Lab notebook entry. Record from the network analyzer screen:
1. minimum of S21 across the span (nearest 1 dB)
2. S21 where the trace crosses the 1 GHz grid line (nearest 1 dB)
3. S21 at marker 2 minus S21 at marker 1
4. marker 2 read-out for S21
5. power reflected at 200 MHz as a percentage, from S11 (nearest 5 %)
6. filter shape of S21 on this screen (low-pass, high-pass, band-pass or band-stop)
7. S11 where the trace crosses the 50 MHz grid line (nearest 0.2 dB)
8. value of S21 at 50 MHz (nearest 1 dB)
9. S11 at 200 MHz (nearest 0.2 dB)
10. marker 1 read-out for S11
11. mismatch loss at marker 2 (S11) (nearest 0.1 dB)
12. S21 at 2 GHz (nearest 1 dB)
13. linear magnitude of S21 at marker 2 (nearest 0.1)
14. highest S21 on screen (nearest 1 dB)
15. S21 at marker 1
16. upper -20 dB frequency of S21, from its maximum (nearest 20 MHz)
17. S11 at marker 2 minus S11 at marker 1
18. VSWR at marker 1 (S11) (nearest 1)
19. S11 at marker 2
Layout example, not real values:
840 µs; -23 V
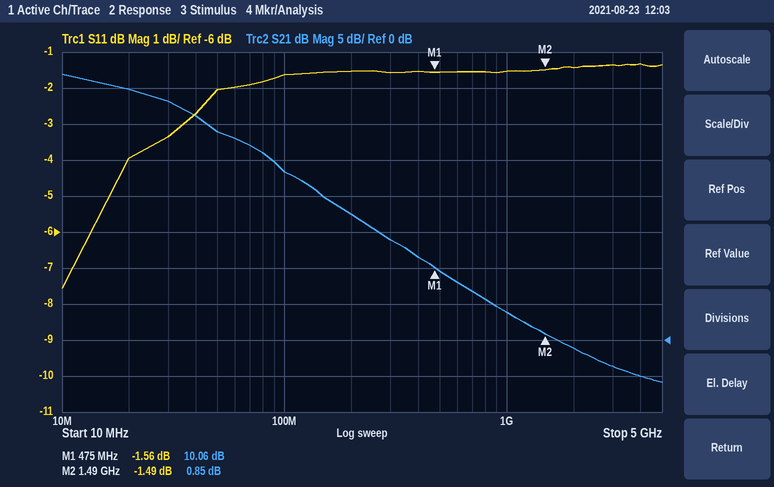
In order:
-6 dB; 4 dB; -9.21 dB; 0.85 dB; 70 %; low-pass; -2.0 dB; 29 dB; -1.6 dB; -1.56 dB; 5.4 dB; -1 dB; 1.1; 37 dB; 10.06 dB; 220 MHz; 0.07 dB; 11; -1.49 dB
